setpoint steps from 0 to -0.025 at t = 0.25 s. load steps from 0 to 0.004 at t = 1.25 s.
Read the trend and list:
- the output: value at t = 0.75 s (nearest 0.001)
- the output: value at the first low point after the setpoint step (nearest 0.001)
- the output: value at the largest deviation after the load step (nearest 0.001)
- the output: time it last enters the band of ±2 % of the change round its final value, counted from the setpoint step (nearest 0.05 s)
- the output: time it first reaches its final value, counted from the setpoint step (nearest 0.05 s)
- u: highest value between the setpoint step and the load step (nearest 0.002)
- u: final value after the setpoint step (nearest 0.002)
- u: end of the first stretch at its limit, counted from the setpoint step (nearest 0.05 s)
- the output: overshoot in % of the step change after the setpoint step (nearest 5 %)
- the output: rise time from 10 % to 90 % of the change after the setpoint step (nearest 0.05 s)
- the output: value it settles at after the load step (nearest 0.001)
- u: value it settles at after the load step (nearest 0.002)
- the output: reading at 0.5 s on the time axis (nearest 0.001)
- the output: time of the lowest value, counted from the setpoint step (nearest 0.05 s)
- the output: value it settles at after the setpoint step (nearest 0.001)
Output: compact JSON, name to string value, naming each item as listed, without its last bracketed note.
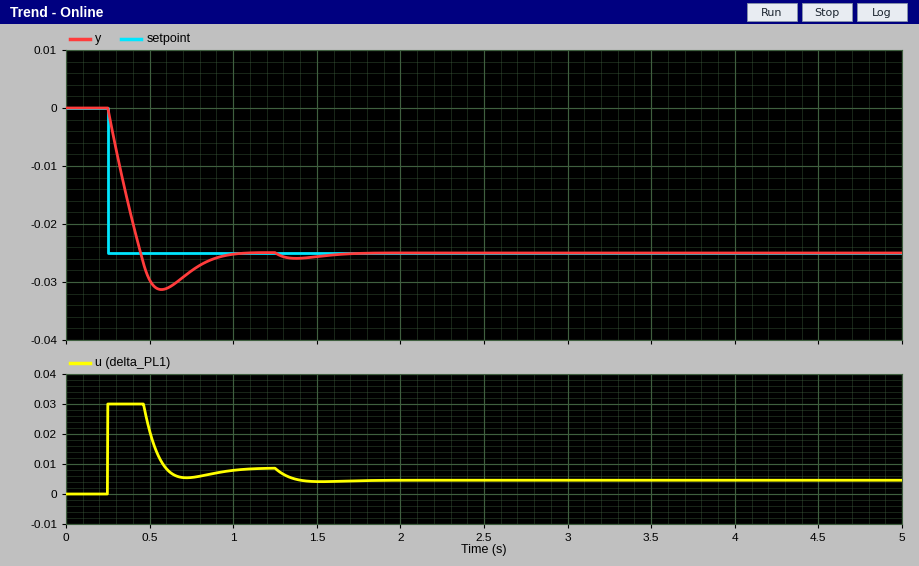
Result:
{"the output: value at t = 0.75 s": "-0.028", "the output: value at the first low point after the setpoint step": "-0.031", "the output: value at the largest deviation after the load step": "-0.026", "the output: time it last enters the band of ±2 % of the change round its final value, counted from the setpoint step": "0.70 s", "the output: time it first reaches its final value, counted from the setpoint step": "0.20 s", "u: highest value between the setpoint step and the load step": "0.030", "u: final value after the setpoint step": "0.008", "u: end of the first stretch at its limit, counted from the setpoint step": "0.20 s", "the output: overshoot in % of the step change after the setpoint step": "25 %", "the output: rise time from 10 % to 90 % of the change after the setpoint step": "0.15 s", "the output: value it settles at after the load step": "-0.025", "u: value it settles at after the load step": "0.004", "the output: reading at 0.5 s on the time axis": "-0.030", "the output: time of the lowest value, counted from the setpoint step": "0.30 s", "the output: value it settles at after the setpoint step": "-0.025"}
